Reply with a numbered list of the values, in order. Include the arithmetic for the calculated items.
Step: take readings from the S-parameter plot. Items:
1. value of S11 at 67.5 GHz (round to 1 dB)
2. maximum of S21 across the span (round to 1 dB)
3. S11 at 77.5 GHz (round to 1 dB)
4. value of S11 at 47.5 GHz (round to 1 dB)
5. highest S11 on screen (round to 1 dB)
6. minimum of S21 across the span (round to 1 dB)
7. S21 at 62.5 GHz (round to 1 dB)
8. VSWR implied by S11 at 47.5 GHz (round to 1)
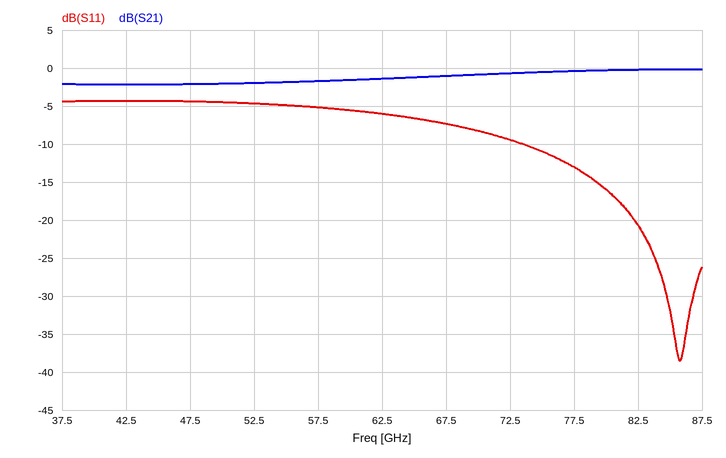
1. -7 dB
2. 0 dB
3. -13 dB
4. -4 dB
5. -4 dB
6. -2 dB
7. -1 dB
8. |Γ| = 10^(-4/20) = 0.6310; VSWR = (1 + 0.6310)/(1 − 0.6310) ≈ 4
